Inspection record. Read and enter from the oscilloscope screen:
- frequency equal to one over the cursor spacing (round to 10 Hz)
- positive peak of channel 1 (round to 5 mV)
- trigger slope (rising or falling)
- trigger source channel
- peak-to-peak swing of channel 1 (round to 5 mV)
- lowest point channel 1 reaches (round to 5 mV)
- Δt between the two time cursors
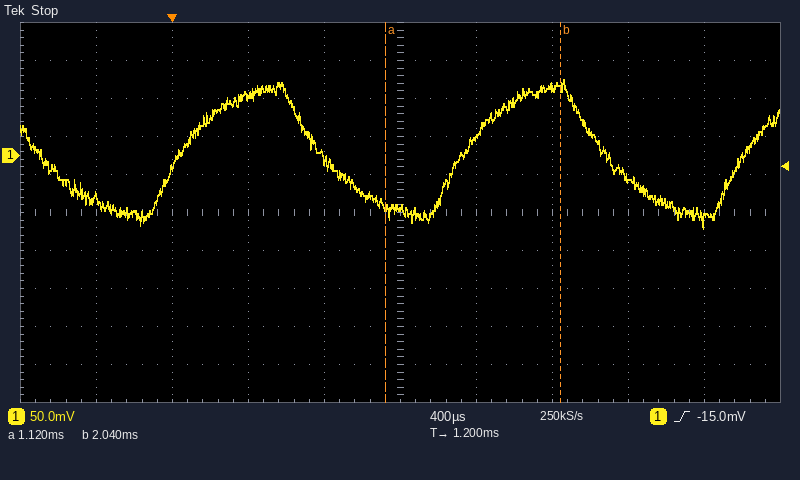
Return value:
1.09 kHz
100 mV
rising
channel 1
195 mV
-95 mV
920 µs
